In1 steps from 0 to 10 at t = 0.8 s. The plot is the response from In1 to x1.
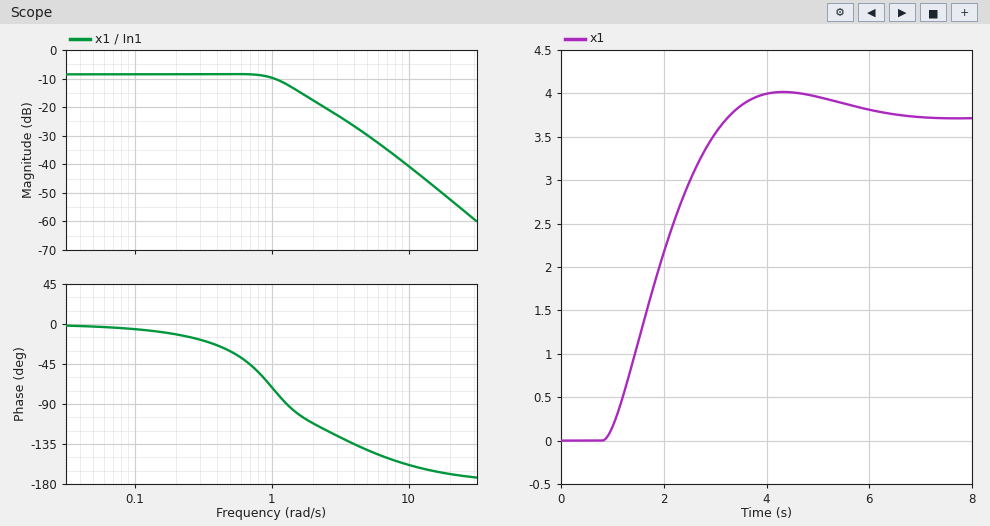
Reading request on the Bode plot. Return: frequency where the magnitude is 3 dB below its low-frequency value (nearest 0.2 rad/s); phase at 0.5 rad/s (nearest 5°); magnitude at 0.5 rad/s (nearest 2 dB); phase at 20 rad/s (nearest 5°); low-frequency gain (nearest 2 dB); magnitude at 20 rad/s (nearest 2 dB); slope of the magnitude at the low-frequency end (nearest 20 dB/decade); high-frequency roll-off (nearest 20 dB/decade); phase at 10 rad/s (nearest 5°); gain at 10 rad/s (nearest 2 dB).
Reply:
1.2 rad/s
-30°
-8 dB
-170°
-8 dB
-52 dB
0 dB/decade
-40 dB/decade
-160°
-40 dB
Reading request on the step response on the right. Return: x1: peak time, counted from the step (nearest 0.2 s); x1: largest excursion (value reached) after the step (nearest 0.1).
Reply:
3.6 s
4.0
